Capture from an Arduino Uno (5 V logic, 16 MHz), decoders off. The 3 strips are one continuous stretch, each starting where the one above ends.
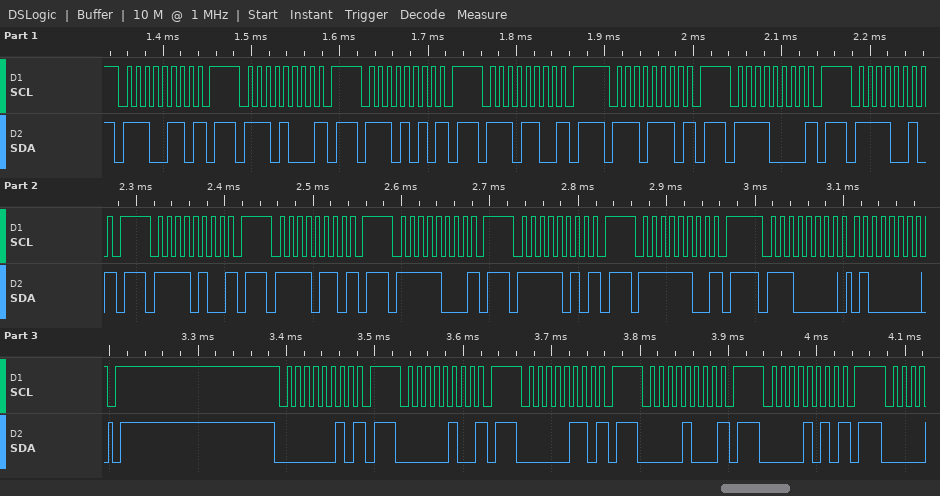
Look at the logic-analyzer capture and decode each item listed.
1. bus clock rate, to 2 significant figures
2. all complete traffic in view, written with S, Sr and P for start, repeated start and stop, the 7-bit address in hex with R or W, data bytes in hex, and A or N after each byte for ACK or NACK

100 kHz
S 73W N P S 74W N P S 75W N P S 76W N P S 77W N P S 78W N P S 79W N P S 7AW N P S 7BW N P S 7CW N P S 7DW N P S 7EW N P S 70W A 40 A P S 01W N P S 02W N P S 03W N P S 04W N P S 05W N P
